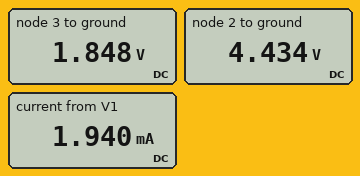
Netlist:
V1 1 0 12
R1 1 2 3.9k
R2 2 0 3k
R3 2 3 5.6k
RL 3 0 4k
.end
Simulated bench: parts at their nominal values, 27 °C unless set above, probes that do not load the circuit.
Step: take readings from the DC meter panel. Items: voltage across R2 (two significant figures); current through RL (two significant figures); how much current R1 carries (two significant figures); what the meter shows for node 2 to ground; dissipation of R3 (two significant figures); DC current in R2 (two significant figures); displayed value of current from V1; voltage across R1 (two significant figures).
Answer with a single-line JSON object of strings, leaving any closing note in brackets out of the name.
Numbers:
{"voltage across R2": "4.4 V", "current through RL": "460 µA", "how much current R1 carries": "1.9 mA", "what the meter shows for node 2 to ground": "4.434 V", "dissipation of R3": "1.2 mW", "DC current in R2": "1.5 mA", "displayed value of current from V1": "1.940 mA", "voltage across R1": "7.6 V"}
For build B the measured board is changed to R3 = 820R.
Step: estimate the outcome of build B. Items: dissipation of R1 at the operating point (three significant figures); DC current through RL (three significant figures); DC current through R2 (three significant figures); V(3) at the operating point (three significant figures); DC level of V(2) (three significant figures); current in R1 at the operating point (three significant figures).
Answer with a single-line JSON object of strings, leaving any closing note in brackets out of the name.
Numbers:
{"dissipation of R1 at the operating point": "17.0 mW", "DC current through RL": "801 µA", "DC current through R2": "1.29 mA", "V(3) at the operating point": "3.20 V", "DC level of V(2)": "3.86 V", "current in R1 at the operating point": "2.09 mA"}
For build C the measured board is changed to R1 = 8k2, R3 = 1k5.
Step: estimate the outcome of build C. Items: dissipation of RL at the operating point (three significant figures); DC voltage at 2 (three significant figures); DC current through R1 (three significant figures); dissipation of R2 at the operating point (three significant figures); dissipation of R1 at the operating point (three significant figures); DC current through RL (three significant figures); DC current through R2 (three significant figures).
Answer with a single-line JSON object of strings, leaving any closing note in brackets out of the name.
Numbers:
{"dissipation of RL at the operating point": "698 µW", "DC voltage at 2": "2.30 V", "DC current through R1": "1.18 mA", "dissipation of R2 at the operating point": "1.76 mW", "dissipation of R1 at the operating point": "11.5 mW", "DC current through RL": "418 µA", "DC current through R2": "766 µA"}
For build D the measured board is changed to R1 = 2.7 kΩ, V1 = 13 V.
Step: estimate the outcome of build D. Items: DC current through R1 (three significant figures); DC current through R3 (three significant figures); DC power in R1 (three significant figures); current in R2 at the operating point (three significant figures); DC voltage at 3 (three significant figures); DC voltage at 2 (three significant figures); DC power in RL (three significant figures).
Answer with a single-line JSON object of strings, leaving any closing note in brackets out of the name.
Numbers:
{"DC current through R1": "2.61 mA", "DC current through R3": "621 µA", "DC power in R1": "18.4 mW", "current in R2 at the operating point": "1.99 mA", "DC voltage at 3": "2.48 V", "DC voltage at 2": "5.96 V", "DC power in RL": "1.54 mW"}
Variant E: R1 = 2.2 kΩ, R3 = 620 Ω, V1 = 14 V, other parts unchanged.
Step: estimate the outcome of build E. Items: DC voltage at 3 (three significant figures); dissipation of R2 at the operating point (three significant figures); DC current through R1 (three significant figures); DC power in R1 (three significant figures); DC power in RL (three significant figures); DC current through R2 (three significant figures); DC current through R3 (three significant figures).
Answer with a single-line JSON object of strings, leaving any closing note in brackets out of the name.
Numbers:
{"DC voltage at 3": "5.49 V", "dissipation of R2 at the operating point": "13.4 mW", "DC current through R1": "3.48 mA", "DC power in R1": "26.7 mW", "DC power in RL": "7.52 mW", "DC current through R2": "2.11 mA", "DC current through R3": "1.37 mA"}
